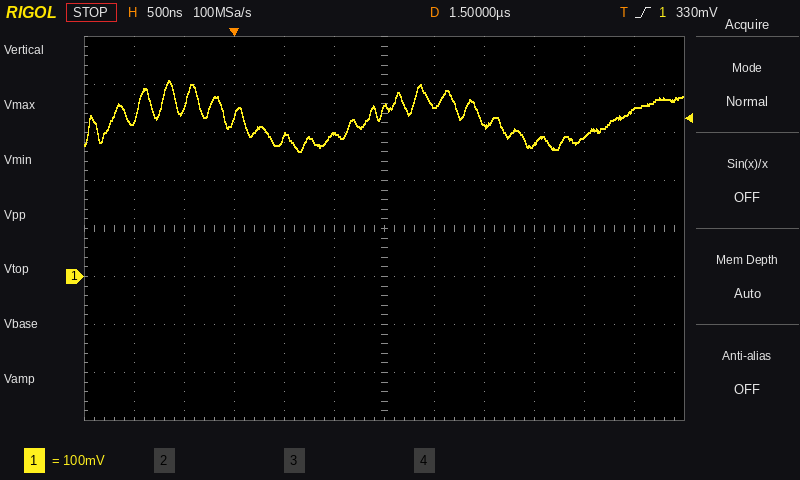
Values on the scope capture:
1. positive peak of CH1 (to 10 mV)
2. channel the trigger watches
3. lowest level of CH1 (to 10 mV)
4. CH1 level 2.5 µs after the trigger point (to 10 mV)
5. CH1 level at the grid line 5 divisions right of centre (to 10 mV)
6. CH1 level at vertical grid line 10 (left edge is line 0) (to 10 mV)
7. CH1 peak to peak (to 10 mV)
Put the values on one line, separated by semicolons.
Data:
410 mV; CH1; 260 mV; 320 mV; 350 mV; 290 mV; 150 mV
